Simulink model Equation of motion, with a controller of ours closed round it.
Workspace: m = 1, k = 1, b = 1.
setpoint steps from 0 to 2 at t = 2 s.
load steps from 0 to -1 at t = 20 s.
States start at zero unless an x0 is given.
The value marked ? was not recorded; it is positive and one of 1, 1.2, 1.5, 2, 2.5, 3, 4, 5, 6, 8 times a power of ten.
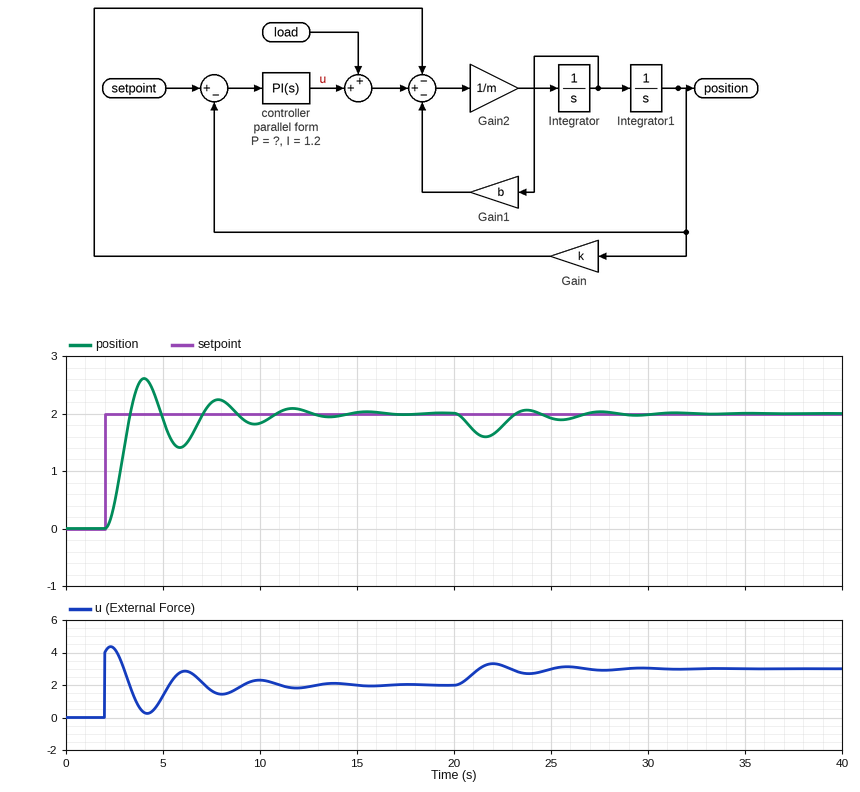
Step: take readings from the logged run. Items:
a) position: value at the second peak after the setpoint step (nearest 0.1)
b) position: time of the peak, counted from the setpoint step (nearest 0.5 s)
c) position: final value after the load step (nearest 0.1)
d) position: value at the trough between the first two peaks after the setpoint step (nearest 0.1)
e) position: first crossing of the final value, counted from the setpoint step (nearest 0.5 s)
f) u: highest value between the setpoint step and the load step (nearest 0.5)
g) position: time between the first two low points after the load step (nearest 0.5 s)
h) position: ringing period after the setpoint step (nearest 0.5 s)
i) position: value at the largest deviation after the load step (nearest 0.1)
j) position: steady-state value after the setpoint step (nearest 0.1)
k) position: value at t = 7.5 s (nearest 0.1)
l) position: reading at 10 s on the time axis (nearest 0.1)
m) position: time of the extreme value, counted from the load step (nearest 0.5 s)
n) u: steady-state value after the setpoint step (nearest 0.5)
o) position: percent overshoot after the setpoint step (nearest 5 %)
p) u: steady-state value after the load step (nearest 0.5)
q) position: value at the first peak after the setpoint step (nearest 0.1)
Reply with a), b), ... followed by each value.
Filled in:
a) 2.2
b) 2.0 s
c) 2.0
d) 1.4
e) 1.5 s
f) 4.5
g) 4.0 s
h) 4.0 s
i) 1.6
j) 2.0
k) 2.2
l) 1.8
m) 1.5 s
n) 2.0
o) 30 %
p) 3.0
q) 2.6
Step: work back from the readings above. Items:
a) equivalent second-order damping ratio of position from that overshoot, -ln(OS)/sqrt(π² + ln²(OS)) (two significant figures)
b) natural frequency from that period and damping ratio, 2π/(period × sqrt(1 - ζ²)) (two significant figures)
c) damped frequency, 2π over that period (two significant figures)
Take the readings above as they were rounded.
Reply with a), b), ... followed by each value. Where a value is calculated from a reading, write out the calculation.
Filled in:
a) ln(0.3) = -1.204; 1.204 / sqrt(9.870 + 1.450) = 0.36
b) 2π / (4 × sqrt(1 - 0.36²)) = 1.7 rad/s
c) 2π / 4 = 1.6 rad/s
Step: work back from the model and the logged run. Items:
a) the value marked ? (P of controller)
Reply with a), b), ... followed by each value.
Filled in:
a) 2
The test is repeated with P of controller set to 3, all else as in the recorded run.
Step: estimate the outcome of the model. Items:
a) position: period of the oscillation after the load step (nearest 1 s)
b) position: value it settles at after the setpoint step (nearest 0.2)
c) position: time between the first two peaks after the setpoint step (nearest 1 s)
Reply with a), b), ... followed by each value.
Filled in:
a) 3 s
b) 2.0
c) 3 s
